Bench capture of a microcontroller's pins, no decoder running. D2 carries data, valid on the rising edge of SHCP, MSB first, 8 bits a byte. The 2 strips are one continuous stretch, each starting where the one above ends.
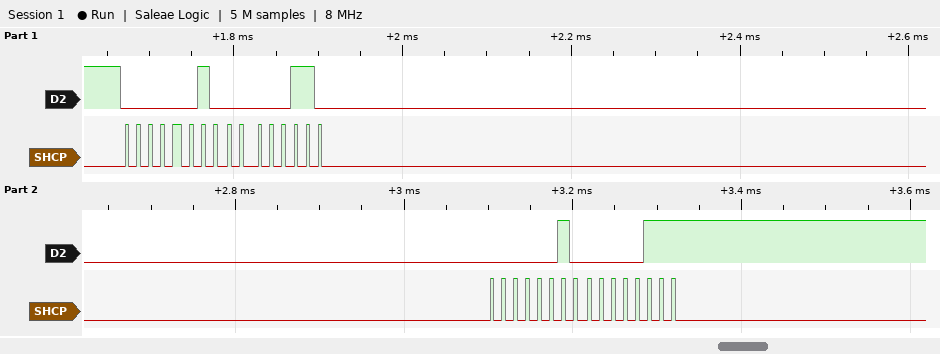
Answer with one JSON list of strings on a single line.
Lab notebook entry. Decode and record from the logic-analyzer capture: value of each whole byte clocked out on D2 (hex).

["02 06 02 07"]
